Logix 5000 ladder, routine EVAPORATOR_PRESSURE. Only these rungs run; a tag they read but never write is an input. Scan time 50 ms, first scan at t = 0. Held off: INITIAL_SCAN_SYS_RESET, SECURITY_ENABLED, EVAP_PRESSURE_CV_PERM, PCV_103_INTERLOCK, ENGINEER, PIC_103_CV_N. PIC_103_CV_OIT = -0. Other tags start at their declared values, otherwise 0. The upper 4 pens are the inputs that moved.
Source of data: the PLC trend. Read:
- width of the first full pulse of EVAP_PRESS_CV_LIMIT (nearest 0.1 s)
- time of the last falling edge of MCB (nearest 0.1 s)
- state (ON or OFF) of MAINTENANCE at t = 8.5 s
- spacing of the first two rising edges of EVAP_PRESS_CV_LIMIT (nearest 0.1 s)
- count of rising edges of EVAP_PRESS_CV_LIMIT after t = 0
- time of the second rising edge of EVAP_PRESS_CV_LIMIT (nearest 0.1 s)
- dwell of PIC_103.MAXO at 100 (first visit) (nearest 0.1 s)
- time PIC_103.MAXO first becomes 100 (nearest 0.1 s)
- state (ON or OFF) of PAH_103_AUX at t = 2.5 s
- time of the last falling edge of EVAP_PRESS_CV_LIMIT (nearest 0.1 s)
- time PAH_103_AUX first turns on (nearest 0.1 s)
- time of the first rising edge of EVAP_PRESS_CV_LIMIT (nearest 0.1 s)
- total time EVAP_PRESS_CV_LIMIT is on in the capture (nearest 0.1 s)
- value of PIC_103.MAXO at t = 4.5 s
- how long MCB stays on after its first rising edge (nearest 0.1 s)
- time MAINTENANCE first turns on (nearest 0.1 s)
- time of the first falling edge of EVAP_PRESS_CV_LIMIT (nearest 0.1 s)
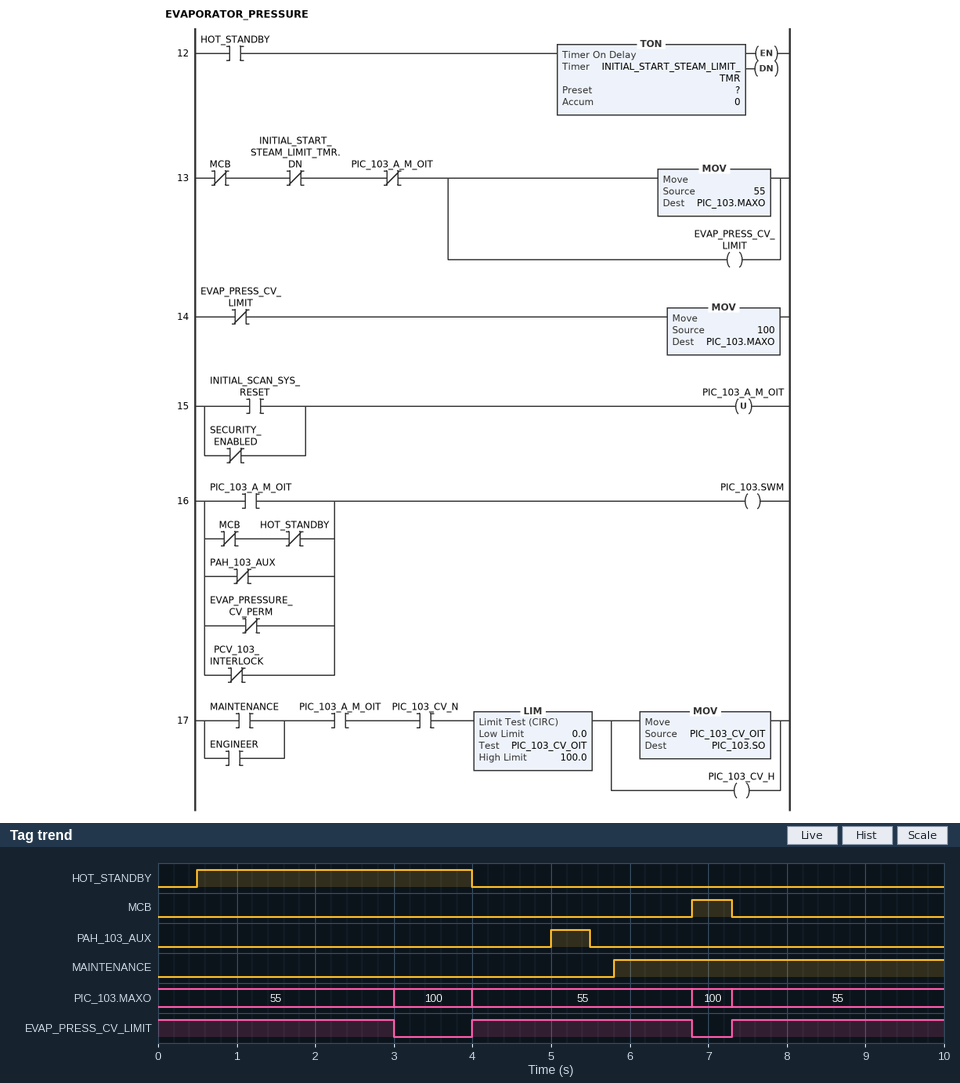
2.8 s
7.3 s
ON
3.3 s
2
7.3 s
1.0 s
3.0 s
OFF
6.8 s
5.0 s
4.0 s
8.5 s
55
0.5 s
5.8 s
3.0 s
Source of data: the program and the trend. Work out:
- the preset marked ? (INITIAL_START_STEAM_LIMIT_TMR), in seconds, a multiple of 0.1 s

2.5 s
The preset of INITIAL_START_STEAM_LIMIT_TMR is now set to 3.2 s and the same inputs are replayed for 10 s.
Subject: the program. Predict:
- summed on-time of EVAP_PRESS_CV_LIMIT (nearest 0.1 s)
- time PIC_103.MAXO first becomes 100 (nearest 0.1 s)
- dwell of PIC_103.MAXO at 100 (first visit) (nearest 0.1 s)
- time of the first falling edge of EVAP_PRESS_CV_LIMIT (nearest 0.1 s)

9.2 s
3.7 s
0.3 s
3.7 s
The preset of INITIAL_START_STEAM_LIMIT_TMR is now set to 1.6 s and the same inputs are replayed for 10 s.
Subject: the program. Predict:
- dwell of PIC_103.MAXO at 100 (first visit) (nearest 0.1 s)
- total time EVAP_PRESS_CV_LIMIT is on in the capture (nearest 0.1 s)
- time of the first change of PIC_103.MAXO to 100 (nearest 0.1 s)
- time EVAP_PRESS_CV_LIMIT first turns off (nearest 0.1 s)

1.9 s
7.6 s
2.1 s
2.1 s
